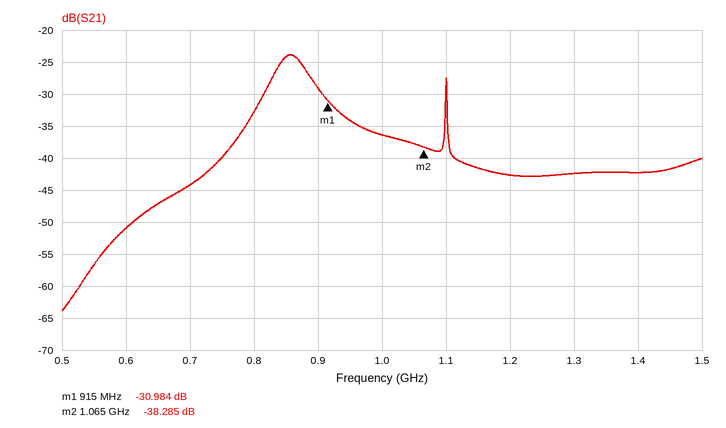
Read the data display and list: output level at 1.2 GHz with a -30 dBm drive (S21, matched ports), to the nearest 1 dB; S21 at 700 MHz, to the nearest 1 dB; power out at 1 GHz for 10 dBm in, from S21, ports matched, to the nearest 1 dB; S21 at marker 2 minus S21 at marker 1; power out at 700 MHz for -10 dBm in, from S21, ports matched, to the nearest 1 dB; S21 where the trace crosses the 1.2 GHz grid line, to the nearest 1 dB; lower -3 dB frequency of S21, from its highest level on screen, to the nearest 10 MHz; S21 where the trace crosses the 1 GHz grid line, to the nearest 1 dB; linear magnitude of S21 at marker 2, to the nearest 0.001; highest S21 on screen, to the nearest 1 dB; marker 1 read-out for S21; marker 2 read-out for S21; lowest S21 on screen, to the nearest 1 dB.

-73 dBm
-44 dB
-26 dBm
-7.301 dB
-54 dBm
-43 dB
830 MHz
-36 dB
0.012
-24 dB
-30.984 dB
-38.285 dB
-64 dB
